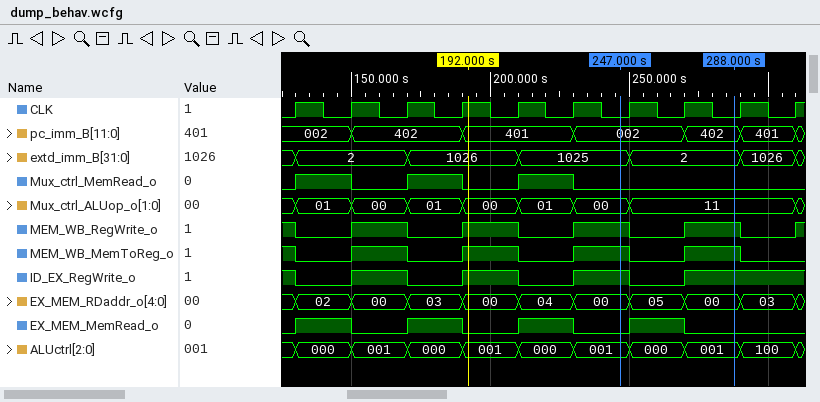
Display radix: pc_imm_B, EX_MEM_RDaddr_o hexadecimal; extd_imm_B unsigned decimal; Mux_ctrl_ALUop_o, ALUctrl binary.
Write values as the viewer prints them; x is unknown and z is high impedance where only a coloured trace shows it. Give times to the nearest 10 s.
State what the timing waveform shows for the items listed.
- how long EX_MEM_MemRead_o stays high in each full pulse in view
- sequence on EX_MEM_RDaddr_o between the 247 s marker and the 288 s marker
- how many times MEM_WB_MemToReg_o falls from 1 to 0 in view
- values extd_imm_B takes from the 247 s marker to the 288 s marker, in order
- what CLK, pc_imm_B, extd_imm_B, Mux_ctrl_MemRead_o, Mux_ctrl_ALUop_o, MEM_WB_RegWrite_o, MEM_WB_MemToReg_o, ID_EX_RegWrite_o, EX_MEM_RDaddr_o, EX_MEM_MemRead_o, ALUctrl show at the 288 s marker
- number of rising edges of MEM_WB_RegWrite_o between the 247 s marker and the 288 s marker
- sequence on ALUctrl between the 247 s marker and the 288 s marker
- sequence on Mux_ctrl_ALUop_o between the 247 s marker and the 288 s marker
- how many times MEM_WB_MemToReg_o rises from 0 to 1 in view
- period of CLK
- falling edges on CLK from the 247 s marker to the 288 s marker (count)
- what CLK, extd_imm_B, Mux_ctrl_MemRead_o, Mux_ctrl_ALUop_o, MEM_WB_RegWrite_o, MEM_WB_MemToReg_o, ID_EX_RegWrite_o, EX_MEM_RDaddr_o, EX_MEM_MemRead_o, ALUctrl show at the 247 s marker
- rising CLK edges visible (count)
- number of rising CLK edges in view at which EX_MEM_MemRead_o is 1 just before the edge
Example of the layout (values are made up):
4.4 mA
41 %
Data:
20 s, 20 s, 20 s, 20 s
00, 05, 00
5
1025, 2
CLK=0, pc_imm_B=402, extd_imm_B=2, Mux_ctrl_MemRead_o=0, Mux_ctrl_ALUop_o=11, MEM_WB_RegWrite_o=1, MEM_WB_MemToReg_o=1, ID_EX_RegWrite_o=1, EX_MEM_RDaddr_o=00, EX_MEM_MemRead_o=0, ALUctrl=001
1
001, 000, 001
00, 11
4
20 s
2
CLK=0, extd_imm_B=1025, Mux_ctrl_MemRead_o=0, Mux_ctrl_ALUop_o=00, MEM_WB_RegWrite_o=1, MEM_WB_MemToReg_o=1, ID_EX_RegWrite_o=1, EX_MEM_RDaddr_o=00, EX_MEM_MemRead_o=0, ALUctrl=001
10
4
